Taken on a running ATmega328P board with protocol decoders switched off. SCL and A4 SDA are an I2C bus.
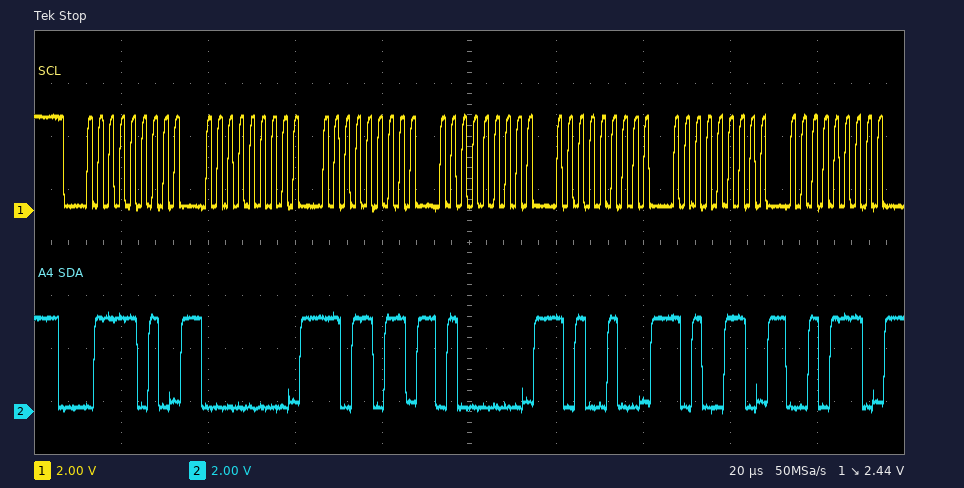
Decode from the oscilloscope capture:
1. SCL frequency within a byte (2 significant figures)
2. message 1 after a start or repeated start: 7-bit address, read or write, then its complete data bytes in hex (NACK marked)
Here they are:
400 kHz
0x3D write: 00 DB 40 A4 A6 2E
